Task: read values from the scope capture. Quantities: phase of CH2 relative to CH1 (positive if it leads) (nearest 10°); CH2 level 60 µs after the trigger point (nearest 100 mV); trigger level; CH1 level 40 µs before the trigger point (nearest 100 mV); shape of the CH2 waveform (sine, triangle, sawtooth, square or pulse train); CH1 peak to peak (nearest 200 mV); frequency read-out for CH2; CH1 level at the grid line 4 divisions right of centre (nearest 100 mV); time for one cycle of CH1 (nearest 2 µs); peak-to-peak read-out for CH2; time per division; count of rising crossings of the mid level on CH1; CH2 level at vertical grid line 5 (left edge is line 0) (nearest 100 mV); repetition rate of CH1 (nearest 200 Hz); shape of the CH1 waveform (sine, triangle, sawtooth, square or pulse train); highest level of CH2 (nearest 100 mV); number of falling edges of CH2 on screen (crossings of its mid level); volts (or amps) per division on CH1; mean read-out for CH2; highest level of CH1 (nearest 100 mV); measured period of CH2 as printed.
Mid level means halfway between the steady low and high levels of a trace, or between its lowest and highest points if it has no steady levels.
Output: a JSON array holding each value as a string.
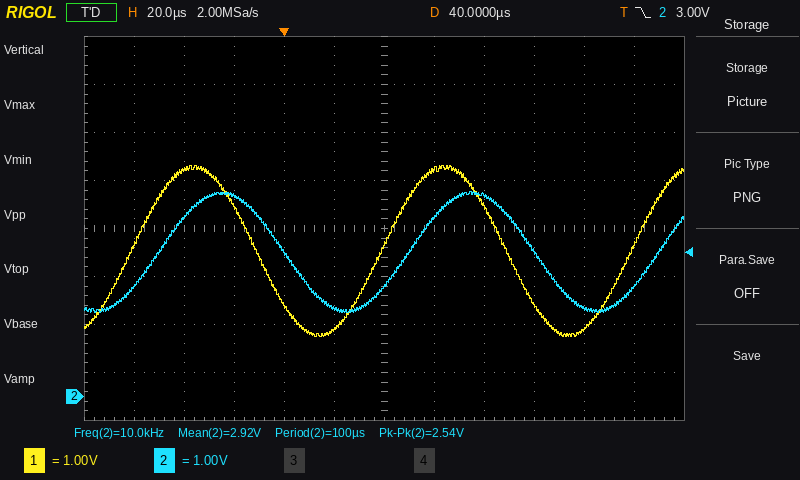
["-40°", "3.7 V", "3.00 V", "4.7 V", "sine", "3.6 V", "10.0 kHz", "1.4 V", "100 µs", "2.54 V", "20 µs", "3", "1.8 V", "10.0 kHz", "sine", "4.3 V", "2", "1 V", "2.92 V", "4.8 V", "100 µs"]
